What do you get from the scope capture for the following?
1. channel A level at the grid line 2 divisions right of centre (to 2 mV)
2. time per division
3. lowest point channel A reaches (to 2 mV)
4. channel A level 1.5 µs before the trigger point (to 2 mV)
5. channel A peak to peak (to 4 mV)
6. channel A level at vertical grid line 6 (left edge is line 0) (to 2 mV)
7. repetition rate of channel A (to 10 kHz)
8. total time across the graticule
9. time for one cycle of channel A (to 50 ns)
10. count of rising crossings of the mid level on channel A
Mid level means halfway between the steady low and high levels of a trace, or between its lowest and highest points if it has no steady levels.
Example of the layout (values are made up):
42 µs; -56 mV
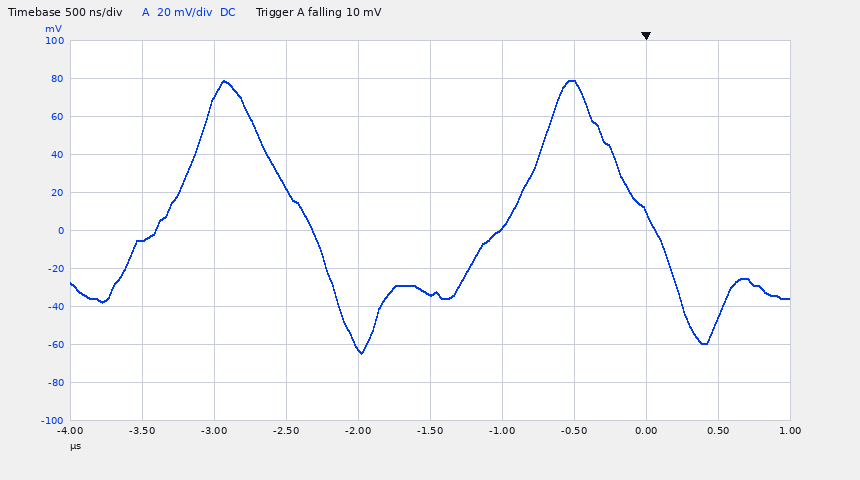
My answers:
78 mV; 500 ns; -64 mV; -34 mV; 144 mV; 2 mV; 420 kHz; 5 µs; 2.40 µs; 2
